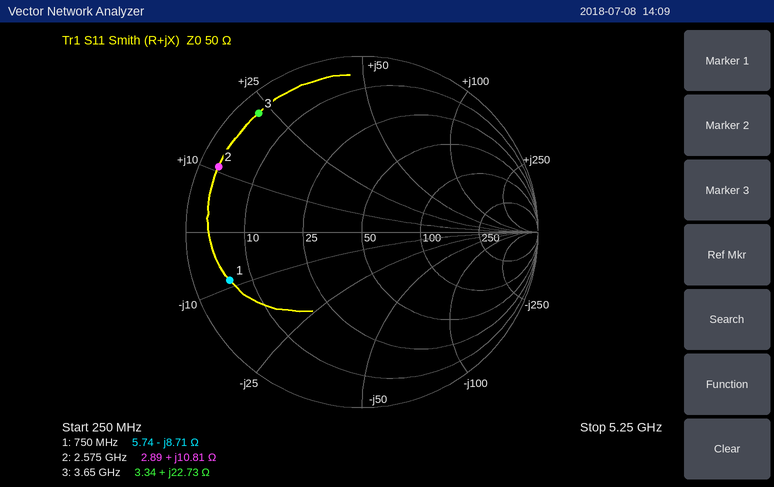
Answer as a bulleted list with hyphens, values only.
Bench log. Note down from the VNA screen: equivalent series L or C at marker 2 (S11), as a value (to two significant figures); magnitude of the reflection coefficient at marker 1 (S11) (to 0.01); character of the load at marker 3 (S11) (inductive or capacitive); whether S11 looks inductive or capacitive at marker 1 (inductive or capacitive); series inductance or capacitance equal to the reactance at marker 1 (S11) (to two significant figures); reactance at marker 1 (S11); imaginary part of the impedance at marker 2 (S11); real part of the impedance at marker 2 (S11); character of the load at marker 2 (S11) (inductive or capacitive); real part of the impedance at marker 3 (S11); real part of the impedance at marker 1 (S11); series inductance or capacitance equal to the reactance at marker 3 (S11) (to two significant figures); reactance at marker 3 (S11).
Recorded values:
- 670 pH
- 0.80
- inductive
- capacitive
- 24 pF
- -8.71 Ω
- +10.81 Ω
- 2.89 Ω
- inductive
- 3.34 Ω
- 5.74 Ω
- 990 pH
- +22.73 Ω
